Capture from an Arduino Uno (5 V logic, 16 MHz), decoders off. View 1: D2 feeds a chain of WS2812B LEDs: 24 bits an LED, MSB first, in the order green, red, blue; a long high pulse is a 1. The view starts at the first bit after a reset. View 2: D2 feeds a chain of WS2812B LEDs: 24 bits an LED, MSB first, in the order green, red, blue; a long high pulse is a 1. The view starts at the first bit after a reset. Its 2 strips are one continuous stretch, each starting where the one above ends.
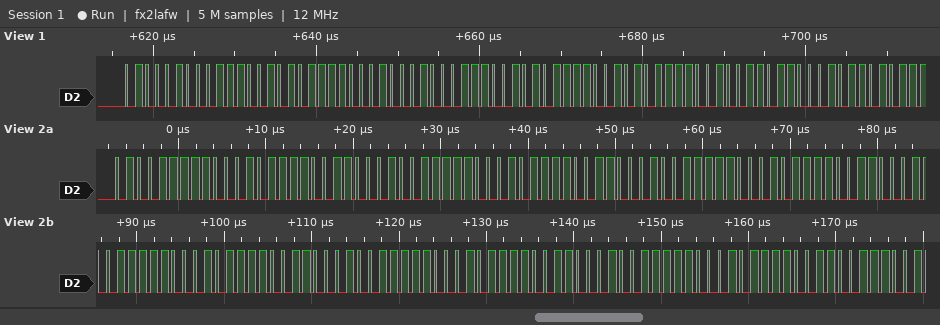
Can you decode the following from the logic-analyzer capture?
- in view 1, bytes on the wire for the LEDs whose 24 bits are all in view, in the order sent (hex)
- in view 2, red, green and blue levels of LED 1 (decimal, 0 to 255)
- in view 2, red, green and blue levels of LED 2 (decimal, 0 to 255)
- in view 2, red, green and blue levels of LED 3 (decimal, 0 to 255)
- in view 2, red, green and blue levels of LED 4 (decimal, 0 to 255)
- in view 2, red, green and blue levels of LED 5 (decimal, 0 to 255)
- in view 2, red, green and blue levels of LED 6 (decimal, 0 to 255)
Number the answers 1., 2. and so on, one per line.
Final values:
1. 44 72 BC 44 72 BC AF 26 C5
2. 139, 79, 204
3. 139, 79, 204
4. 139, 79, 204
5. 139, 79, 204
6. 139, 79, 204
7. 139, 79, 204
